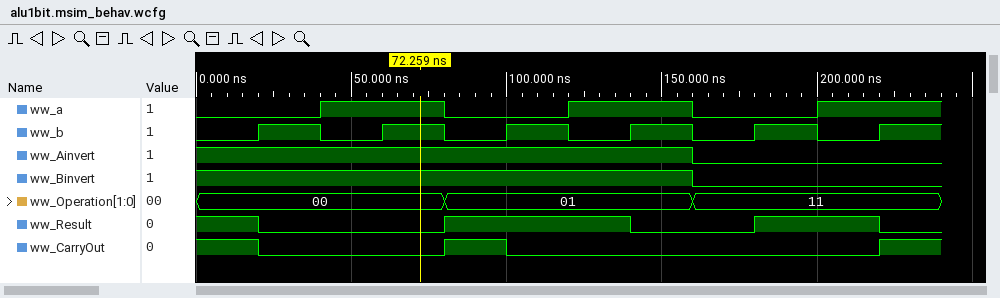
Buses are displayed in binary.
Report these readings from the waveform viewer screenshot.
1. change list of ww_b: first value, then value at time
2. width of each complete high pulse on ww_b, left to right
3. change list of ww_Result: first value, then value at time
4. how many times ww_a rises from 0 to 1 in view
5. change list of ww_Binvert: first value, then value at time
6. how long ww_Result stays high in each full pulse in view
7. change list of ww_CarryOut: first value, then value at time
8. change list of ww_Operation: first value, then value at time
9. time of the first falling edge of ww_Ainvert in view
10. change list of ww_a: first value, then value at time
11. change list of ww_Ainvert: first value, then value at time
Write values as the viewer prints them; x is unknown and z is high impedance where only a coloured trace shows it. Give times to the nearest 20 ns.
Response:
0, 1 at 20 ns, 0 at 40 ns, 1 at 60 ns, 0 at 80 ns, 1 at 100 ns, 0 at 120 ns, 1 at 140 ns, 0 at 160 ns, 1 at 180 ns, 0 at 200 ns, 1 at 220 ns
20 ns, 20 ns, 20 ns, 20 ns, 20 ns
1, 0 at 20 ns, 1 at 80 ns, 0 at 140 ns, 1 at 180 ns, 0 at 220 ns
3
1, 0 at 160 ns
60 ns, 40 ns
1, 0 at 20 ns, 1 at 80 ns, 0 at 100 ns, 1 at 220 ns
00, 01 at 80 ns, 11 at 160 ns
160 ns
0, 1 at 40 ns, 0 at 80 ns, 1 at 120 ns, 0 at 160 ns, 1 at 200 ns
1, 0 at 160 ns
